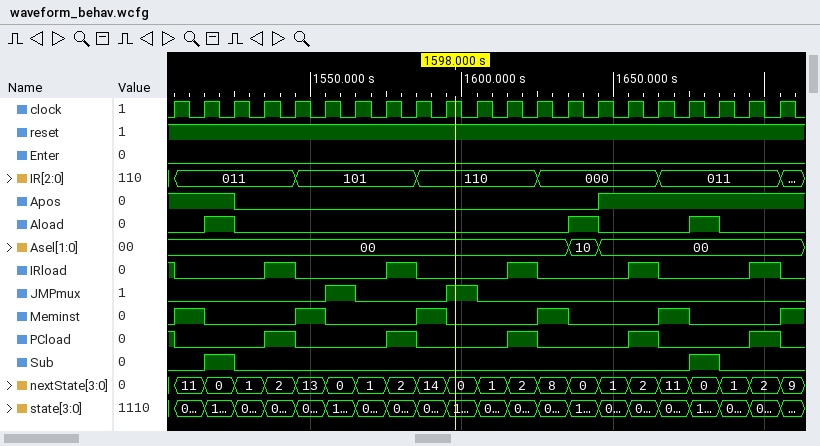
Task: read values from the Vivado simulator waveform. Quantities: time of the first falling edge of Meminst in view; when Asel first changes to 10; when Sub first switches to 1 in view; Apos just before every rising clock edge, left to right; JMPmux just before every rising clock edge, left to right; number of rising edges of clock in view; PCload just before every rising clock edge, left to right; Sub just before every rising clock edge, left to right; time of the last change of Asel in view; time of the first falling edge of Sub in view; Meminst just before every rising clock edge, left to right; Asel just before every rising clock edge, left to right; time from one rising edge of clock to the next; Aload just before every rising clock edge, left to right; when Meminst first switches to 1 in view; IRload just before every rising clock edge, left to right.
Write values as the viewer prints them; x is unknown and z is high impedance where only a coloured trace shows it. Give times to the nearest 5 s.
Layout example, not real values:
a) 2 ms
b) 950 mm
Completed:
a) 1515 s
b) 1635 s
c) 1515 s
d) 1 1 1 0 0 0 0 0 0 0 0 0 0 0 0 1 1 1 1 1 1
e) 0 0 0 0 0 0 1 0 0 0 1 0 0 0 0 0 0 0 0 0 0
f) 21
g) 1 0 0 0 1 0 0 0 1 0 0 0 1 0 0 0 1 0 0 0 1
h) 0 0 1 0 0 0 0 0 0 0 0 0 0 0 0 0 0 0 1 0 0
i) 1645 s
j) 1525 s
k) 0 1 0 0 0 1 0 0 0 1 0 0 0 1 0 0 0 1 0 0 0
l) 00, 00, 00, 00, 00, 00, 00, 00, 00, 00, 00, 00, 00, 00, 10, 00, 00, 00, 00, 00, 00
m) 10 s
n) 0 0 1 0 0 0 0 0 0 0 0 0 0 0 1 0 0 0 1 0 0
o) 1505 s
p) 1 0 0 0 1 0 0 0 1 0 0 0 1 0 0 0 1 0 0 0 1
